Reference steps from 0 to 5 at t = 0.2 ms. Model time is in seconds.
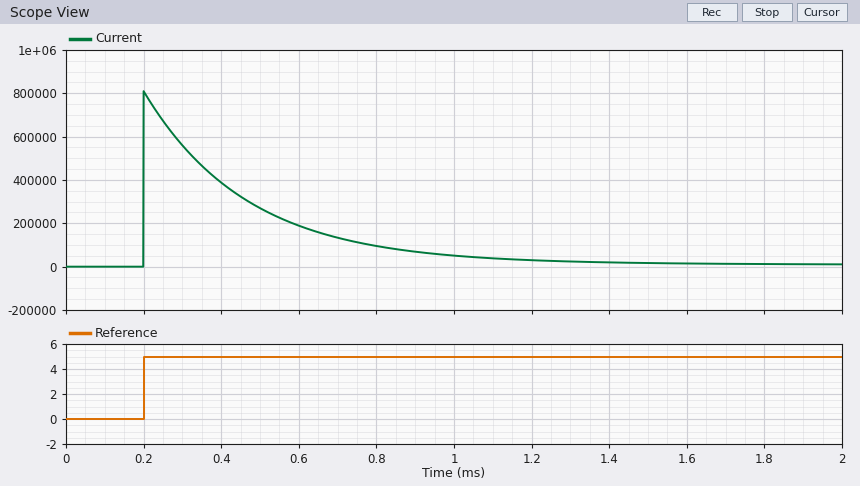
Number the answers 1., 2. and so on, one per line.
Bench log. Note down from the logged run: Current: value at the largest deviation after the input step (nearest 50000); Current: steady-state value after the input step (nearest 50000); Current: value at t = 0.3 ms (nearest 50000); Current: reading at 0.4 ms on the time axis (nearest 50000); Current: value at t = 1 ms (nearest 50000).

1. 800000
2. 0
3. 550000
4. 400000
5. 50000
